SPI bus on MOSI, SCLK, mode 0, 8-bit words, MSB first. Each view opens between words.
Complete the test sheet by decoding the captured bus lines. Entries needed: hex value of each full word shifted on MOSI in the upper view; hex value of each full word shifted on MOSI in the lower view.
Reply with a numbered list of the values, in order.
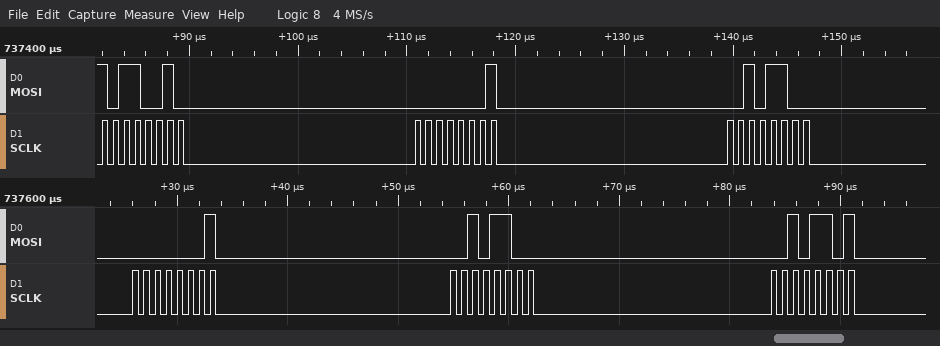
1. B2, 01, 2C
2. 01, 2C, 2D
